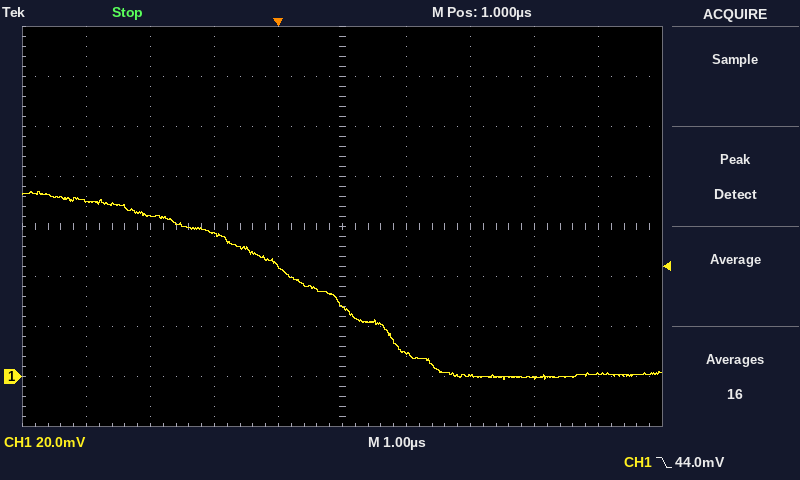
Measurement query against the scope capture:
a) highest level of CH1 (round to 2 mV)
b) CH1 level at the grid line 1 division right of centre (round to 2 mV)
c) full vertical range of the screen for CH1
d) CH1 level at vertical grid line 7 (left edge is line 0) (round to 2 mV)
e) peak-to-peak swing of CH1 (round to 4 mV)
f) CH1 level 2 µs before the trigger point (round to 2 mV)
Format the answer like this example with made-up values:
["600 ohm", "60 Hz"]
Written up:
["74 mV", "10 mV", "160 mV", "0 mV", "76 mV", "64 mV"]
